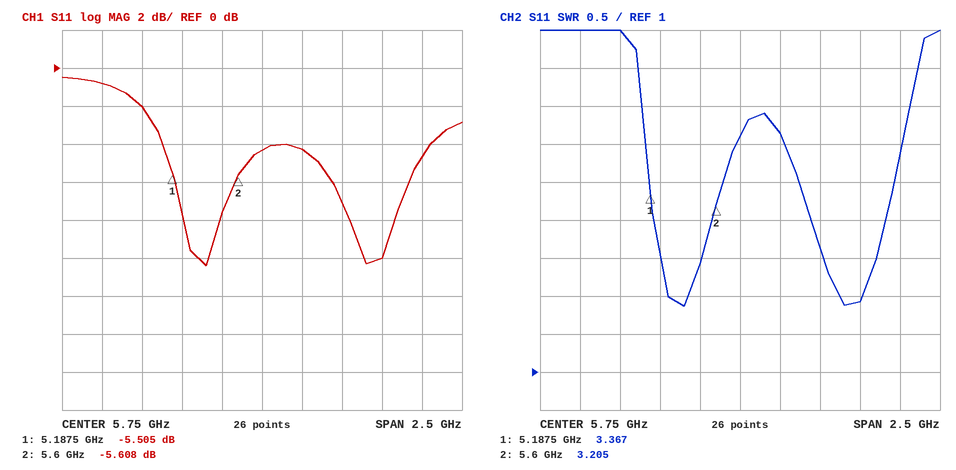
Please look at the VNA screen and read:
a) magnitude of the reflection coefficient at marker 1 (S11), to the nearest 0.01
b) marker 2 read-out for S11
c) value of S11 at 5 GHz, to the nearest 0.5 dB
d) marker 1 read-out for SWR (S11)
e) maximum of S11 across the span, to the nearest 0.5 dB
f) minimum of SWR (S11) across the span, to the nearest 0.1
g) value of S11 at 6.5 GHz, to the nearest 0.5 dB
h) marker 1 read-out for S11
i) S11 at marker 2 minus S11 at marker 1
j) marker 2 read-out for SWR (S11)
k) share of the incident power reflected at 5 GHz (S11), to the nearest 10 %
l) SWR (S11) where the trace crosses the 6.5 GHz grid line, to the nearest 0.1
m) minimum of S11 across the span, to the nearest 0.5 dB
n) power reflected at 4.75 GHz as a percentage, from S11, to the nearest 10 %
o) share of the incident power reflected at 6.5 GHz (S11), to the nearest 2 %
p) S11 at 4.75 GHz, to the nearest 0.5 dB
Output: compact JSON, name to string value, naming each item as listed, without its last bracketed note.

{"magnitude of the reflection coefficient at marker 1 (S11), to the nearest 0.01": "0.53", "marker 2 read-out for S11": "-5.608 dB", "value of S11 at 5 GHz, to the nearest 0.5 dB": "-2.0 dB", "marker 1 read-out for SWR": "3.367", "maximum of S11 across the span, to the nearest 0.5 dB": "-0.5 dB", "minimum of SWR (S11) across the span, to the nearest 0.1": "1.9", "value of S11 at 6.5 GHz, to the nearest 0.5 dB": "-10.0 dB", "marker 1 read-out for S11": "-5.505 dB", "S11 at marker 2 minus S11 at marker 1": "-0.103 dB", "marker 2 read-out for SWR": "3.205", "share of the incident power reflected at 5 GHz (S11), to the nearest 10 %": "60 %", "SWR (S11) where the trace crosses the 6.5 GHz grid line, to the nearest 0.1": "1.9", "minimum of S11 across the span, to the nearest 0.5 dB": "-10.5 dB", "power reflected at 4.75 GHz as a percentage, from S11, to the nearest 10 %": "80 %", "share of the incident power reflected at 6.5 GHz (S11), to the nearest 2 %": "10 %", "S11 at 4.75 GHz, to the nearest 0.5 dB": "-1.0 dB"}
